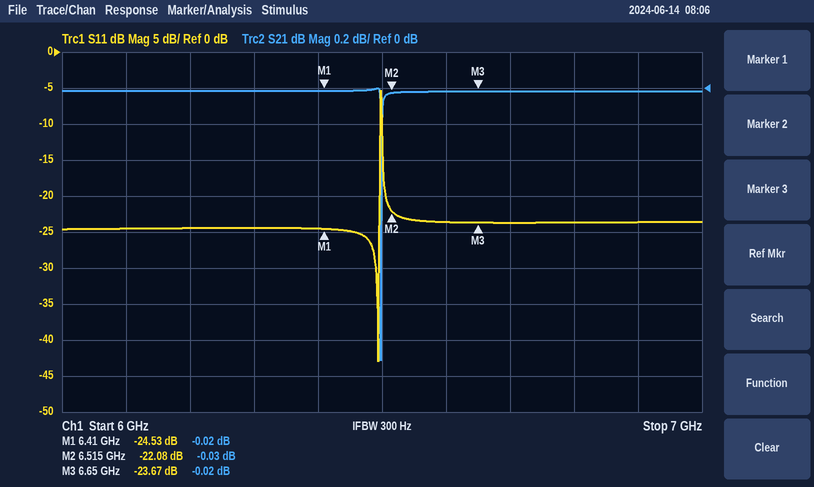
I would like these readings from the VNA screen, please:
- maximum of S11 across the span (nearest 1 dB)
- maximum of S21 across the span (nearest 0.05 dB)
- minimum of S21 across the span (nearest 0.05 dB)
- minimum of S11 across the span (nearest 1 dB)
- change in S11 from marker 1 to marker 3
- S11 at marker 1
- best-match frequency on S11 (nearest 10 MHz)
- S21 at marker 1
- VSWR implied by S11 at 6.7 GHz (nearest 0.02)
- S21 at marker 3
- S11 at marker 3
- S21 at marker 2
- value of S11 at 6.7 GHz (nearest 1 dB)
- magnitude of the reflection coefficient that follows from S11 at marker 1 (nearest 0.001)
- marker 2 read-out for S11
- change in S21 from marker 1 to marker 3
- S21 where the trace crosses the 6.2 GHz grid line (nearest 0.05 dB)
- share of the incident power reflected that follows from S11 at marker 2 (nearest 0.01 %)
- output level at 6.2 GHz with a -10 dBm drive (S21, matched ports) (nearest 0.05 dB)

-5 dB
0.00 dB
-1.50 dB
-43 dB
0.86 dB
-24.53 dB
6.49 GHz
-0.02 dB
1.14
-0.02 dB
-23.67 dB
-0.03 dB
-24 dB
0.059
-22.08 dB
0.00 dB
0.00 dB
0.62 %
-10.00 dBm
